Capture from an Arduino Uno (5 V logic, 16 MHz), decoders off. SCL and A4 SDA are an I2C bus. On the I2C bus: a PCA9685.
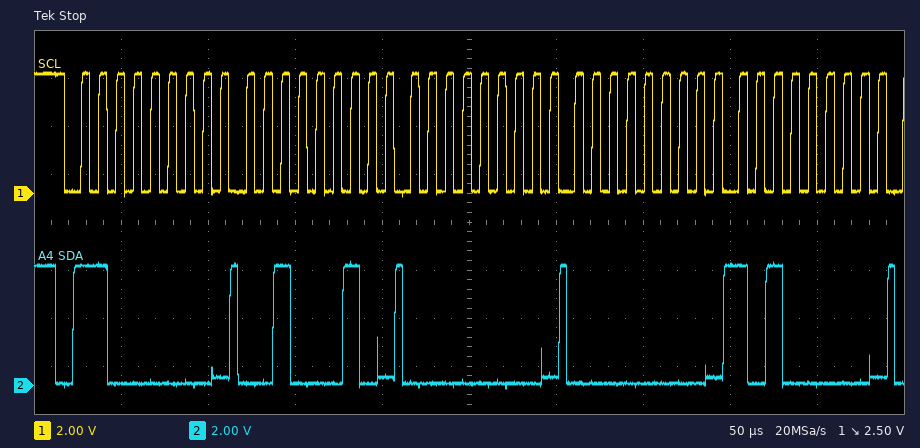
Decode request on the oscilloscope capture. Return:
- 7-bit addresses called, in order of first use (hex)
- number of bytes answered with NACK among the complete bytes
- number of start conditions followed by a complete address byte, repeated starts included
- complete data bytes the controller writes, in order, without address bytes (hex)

0x60
0
1
22 00 00 A0
